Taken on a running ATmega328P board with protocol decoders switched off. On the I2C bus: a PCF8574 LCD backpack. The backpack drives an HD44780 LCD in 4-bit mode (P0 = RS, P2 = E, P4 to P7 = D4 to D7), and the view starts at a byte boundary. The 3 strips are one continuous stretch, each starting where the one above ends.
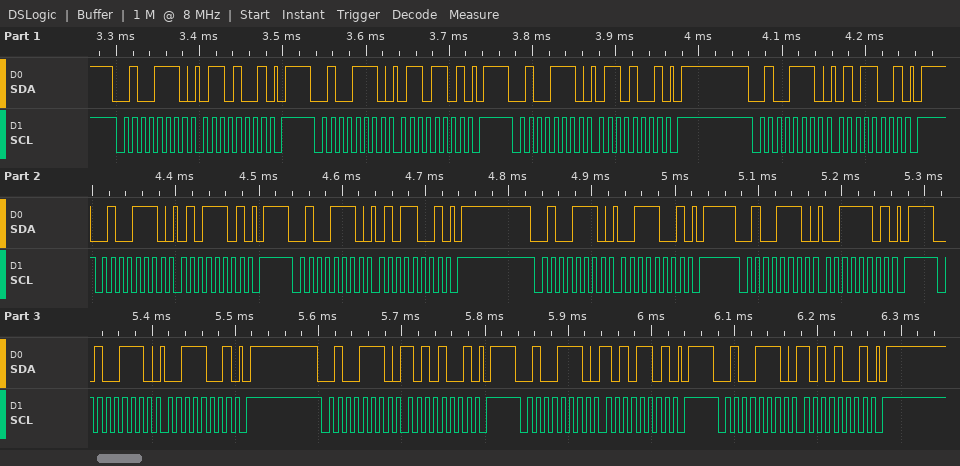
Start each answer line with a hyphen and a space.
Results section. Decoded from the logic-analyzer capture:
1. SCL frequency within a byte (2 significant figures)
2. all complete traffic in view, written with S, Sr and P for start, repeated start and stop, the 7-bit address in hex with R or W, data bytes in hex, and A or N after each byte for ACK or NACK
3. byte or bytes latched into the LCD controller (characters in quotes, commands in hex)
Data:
- 100 kHz
- S 27W A 69 A P S 27W A 6D A P S 27W A 69 A P S 27W A 59 A P S 27W A 5D A P S 27W A 59 A P S 27W A 39 A P S 27W A 3D A P S 27W A 39 A P S 27W A A9 A P S 27W A AD A P S 27W A A9 A P
- 'e' ':'
